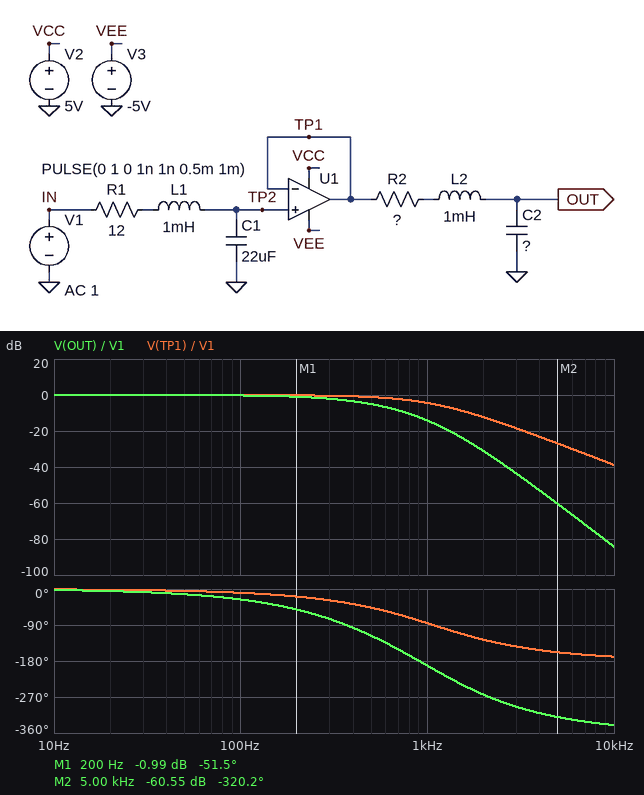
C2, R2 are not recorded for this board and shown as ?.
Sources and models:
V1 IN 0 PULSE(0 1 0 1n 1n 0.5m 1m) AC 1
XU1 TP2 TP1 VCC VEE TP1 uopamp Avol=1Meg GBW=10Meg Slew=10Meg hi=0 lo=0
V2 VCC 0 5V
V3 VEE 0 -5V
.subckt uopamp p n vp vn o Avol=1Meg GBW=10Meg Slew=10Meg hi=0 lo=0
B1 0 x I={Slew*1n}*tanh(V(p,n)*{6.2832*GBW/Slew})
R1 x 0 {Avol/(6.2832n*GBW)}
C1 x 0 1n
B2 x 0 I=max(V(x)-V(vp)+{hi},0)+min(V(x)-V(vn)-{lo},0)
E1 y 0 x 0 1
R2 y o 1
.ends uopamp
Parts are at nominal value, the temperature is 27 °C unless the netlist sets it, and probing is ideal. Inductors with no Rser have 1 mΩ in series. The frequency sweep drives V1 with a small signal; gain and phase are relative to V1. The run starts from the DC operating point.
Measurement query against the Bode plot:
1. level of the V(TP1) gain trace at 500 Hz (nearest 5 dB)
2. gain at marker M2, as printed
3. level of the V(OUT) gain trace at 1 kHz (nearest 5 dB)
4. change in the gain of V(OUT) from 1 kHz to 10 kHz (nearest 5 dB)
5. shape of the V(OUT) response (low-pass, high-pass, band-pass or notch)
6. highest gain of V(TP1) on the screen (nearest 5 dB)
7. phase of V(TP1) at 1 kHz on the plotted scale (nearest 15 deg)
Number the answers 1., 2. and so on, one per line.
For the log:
1. 0 dB
2. -60.55 dB
3. -15 dB
4. -70 dB
5. low-pass
6. 0 dB
7. -90 deg
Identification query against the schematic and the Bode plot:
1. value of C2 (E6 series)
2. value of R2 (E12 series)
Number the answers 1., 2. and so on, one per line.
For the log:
1. 47 µF
2. 10 Ω
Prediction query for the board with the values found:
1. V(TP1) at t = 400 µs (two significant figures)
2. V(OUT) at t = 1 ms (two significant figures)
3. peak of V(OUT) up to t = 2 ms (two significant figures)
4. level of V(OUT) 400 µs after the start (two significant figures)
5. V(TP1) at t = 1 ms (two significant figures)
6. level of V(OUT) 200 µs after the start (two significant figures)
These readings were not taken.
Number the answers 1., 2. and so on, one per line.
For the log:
1. 800 mV
2. 490 mV
3. 620 mV
4. 190 mV
5. 100 mV
6. 27 mV
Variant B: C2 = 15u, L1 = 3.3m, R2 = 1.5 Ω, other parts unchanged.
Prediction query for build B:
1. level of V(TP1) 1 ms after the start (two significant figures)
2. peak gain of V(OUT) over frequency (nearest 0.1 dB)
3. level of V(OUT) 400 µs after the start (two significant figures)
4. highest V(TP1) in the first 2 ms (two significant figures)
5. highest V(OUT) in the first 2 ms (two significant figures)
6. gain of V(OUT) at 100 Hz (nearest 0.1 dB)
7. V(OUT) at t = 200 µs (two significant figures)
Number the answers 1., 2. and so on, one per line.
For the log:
1. 380 mV
2. 2.5 dB
3. 430 mV
4. 890 mV
5. 1.2 V
6. 0.2 dB
7. 45 mV
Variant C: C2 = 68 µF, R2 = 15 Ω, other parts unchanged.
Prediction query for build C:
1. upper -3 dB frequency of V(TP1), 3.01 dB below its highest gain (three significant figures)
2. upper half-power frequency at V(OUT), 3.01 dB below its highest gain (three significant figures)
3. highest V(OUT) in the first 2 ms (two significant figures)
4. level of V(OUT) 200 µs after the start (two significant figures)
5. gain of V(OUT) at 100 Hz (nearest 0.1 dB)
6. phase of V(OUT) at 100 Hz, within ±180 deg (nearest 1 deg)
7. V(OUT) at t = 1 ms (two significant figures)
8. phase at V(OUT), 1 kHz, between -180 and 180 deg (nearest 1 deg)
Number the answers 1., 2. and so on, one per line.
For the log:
1. 813 Hz
2. 162 Hz
3. 480 mV
4. 16 mV
5. -1.4 dB
6. -43 deg
7. 320 mV
8. 170 deg
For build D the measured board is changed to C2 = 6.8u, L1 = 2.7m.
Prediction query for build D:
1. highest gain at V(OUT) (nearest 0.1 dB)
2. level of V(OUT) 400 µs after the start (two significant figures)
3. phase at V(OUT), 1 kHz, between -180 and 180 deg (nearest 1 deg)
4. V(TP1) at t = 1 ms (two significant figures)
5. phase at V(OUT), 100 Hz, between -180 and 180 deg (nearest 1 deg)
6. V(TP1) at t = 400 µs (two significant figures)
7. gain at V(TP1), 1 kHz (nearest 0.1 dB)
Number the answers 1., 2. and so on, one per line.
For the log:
1. 1.1 dB
2. 500 mV
3. -159 deg
4. 280 mV
5. -12 deg
6. 660 mV
7. -6.6 dB
